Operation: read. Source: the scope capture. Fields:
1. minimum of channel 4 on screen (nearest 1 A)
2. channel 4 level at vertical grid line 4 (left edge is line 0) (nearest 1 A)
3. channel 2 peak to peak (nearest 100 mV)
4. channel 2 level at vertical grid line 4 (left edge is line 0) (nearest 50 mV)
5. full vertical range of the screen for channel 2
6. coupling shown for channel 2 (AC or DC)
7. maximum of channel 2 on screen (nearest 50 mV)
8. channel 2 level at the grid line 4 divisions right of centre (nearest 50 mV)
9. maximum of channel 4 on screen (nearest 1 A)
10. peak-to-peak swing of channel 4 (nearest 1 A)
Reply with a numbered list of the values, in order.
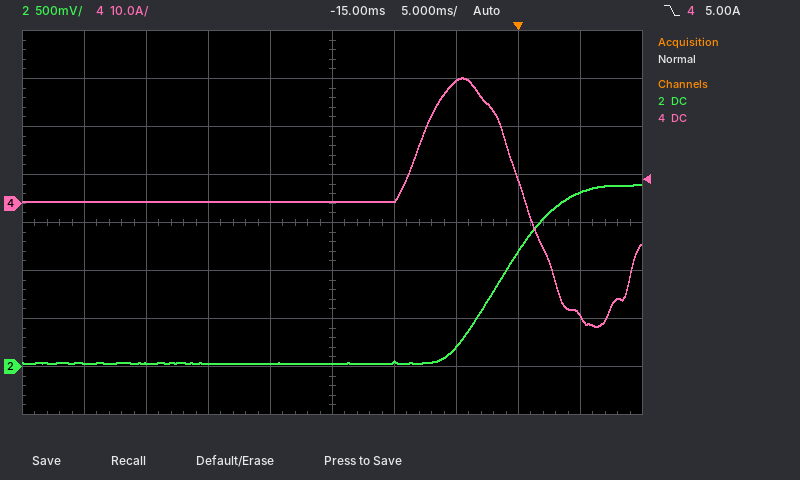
1. -26 A
2. 0 A
3. 1.90 V
4. 50 mV
5. 4 V
6. DC
7. 1.90 V
8. 1.80 V
9. 26 A
10. 52 A
